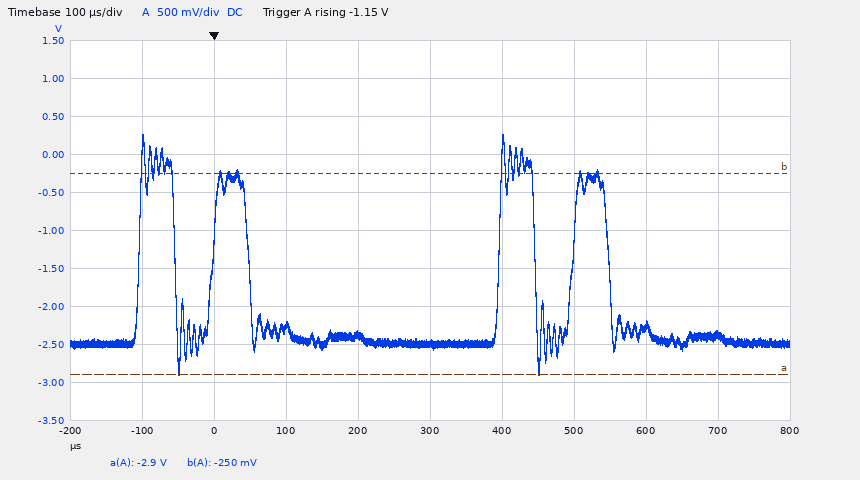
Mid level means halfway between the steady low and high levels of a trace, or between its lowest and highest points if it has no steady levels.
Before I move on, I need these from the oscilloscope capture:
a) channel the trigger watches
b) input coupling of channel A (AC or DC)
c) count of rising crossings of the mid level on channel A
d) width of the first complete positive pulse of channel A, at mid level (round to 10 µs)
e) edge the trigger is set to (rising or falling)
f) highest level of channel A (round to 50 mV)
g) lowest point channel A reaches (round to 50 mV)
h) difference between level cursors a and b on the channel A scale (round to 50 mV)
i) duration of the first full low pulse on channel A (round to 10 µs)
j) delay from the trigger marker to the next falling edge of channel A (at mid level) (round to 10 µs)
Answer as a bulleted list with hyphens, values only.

- channel A
- DC
- 4
- 50 µs
- rising
- 250 mV
- -2.90 V
- 2.65 V
- 50 µs
- 50 µs
